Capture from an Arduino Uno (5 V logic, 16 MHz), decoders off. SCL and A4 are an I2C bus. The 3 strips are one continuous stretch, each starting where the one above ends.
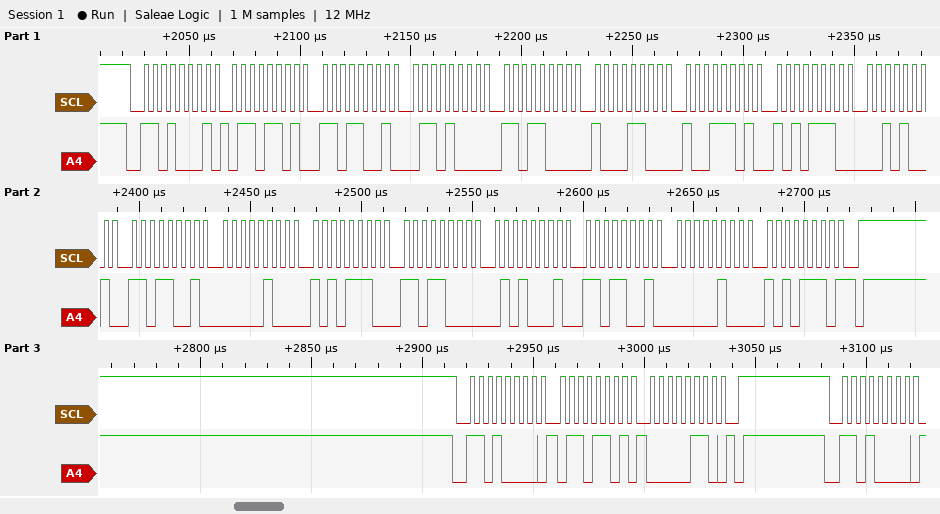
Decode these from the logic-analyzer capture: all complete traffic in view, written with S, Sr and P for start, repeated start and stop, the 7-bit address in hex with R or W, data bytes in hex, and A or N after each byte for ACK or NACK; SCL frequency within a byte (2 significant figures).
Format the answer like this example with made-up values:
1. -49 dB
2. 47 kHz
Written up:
1. S 68R A 6D A D9 A 68 A D8 A 8C A 9D A AE A 29 A D9 A 04 A AE A D8 A 51 A D9 A 04 A AE N P S 68W A 6D A 06 A P S 68W A
2. 250 kHz
